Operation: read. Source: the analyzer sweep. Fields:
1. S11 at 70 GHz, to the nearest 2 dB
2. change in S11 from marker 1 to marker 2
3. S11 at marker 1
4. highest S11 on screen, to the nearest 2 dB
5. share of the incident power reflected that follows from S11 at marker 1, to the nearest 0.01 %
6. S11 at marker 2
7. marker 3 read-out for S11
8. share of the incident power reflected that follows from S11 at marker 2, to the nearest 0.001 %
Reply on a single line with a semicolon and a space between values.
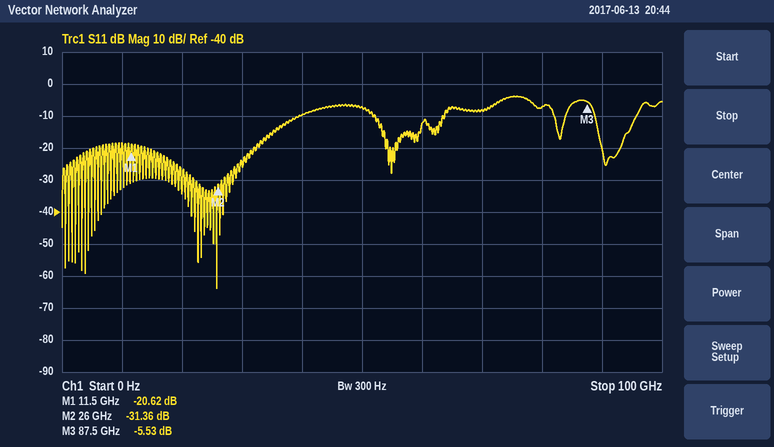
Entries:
-8 dB; -10.74 dB; -20.62 dB; -4 dB; 0.87 %; -31.36 dB; -5.53 dB; 0.073 %
